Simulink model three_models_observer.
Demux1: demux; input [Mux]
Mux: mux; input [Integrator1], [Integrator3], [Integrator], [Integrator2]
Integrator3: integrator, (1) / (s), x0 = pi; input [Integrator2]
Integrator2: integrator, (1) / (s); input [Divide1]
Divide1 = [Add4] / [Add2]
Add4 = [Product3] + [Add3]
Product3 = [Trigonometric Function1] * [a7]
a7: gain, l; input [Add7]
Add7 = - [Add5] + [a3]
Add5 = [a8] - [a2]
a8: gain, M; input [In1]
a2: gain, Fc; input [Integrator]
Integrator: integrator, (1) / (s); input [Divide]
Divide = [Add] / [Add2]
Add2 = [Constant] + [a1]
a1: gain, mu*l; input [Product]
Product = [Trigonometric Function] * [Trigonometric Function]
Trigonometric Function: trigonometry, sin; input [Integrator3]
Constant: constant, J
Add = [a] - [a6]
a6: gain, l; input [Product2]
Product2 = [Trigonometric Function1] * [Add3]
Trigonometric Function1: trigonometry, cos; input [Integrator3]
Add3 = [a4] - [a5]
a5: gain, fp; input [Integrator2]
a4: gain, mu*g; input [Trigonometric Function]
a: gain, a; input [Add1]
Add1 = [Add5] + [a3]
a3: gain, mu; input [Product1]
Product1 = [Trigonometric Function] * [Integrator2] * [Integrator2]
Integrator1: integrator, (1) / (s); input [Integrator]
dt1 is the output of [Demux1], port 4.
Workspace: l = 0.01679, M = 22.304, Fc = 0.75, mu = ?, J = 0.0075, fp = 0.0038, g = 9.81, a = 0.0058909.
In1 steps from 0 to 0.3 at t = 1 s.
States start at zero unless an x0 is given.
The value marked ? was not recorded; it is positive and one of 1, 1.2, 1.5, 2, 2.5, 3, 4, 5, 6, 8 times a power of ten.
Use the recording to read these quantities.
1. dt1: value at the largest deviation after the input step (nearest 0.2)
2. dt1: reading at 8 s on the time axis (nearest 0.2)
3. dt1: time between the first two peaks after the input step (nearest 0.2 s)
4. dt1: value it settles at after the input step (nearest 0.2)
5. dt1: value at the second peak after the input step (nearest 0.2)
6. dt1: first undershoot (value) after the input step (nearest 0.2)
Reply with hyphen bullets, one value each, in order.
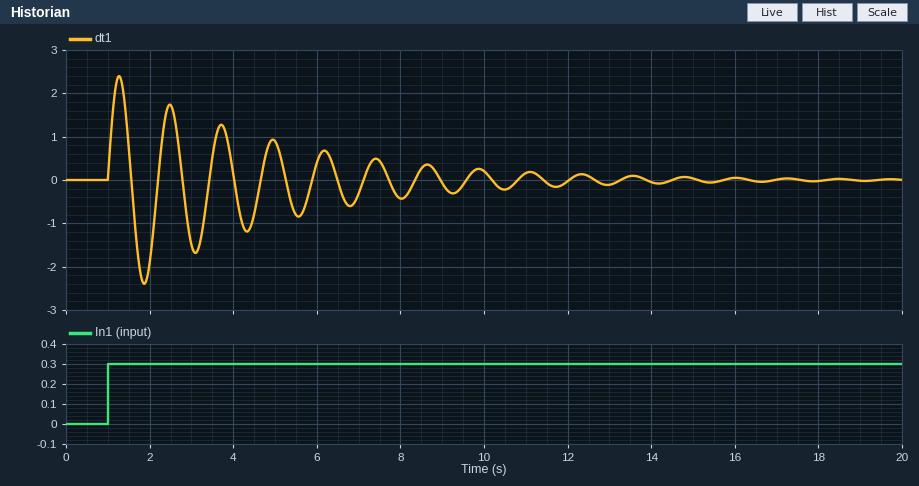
- 2.4
- -0.4
- 1.2 s
- 0.0
- 1.8
- -2.4
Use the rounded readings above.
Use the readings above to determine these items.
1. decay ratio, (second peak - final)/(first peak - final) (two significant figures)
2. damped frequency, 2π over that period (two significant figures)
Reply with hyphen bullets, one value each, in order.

- 0.75
- 5.2 rad/s
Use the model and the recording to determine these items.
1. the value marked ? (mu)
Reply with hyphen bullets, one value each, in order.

- 0.02
